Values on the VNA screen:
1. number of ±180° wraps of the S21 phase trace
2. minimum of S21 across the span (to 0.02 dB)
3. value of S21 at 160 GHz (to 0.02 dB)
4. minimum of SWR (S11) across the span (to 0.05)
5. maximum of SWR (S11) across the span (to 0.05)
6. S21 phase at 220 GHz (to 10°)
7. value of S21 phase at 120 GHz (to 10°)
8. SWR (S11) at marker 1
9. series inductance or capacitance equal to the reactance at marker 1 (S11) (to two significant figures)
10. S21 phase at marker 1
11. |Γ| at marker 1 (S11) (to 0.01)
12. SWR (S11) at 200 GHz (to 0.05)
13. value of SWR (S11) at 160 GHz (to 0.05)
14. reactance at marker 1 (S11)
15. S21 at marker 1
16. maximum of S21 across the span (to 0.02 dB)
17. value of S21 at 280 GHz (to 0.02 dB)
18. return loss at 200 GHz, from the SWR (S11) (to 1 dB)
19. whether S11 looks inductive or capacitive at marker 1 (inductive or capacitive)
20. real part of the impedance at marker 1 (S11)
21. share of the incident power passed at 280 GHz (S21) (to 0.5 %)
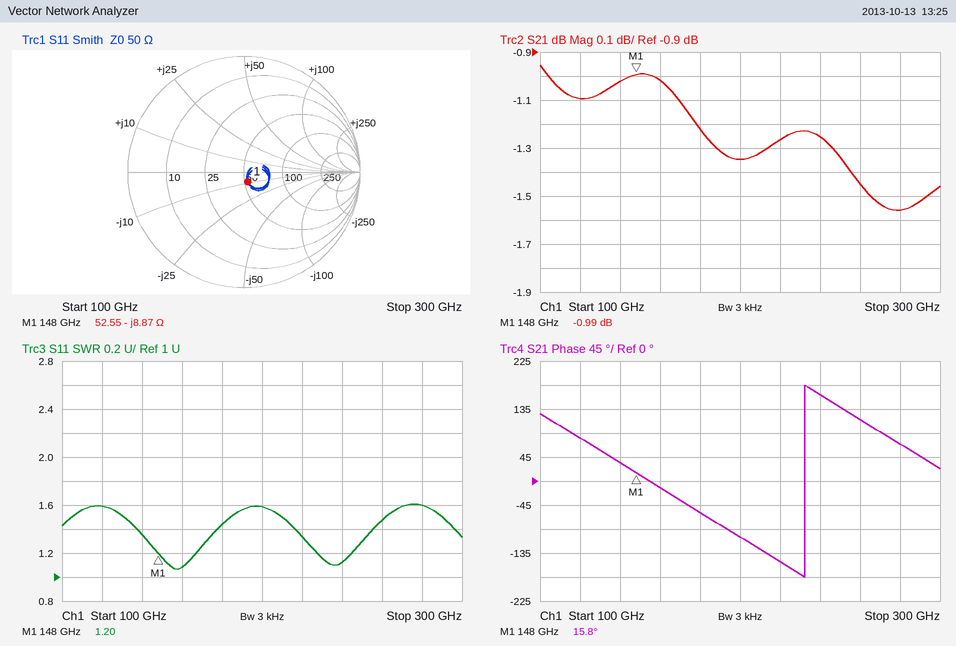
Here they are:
1
-1.56 dB
-1.02 dB
1.05
1.60
-150°
80°
1.20
120 fF
15.8°
0.09
1.60
1.10
-8.87 Ω
-0.99 dB
-0.96 dB
-1.56 dB
13 dB
capacitive
52.55 Ω
70.0 %
